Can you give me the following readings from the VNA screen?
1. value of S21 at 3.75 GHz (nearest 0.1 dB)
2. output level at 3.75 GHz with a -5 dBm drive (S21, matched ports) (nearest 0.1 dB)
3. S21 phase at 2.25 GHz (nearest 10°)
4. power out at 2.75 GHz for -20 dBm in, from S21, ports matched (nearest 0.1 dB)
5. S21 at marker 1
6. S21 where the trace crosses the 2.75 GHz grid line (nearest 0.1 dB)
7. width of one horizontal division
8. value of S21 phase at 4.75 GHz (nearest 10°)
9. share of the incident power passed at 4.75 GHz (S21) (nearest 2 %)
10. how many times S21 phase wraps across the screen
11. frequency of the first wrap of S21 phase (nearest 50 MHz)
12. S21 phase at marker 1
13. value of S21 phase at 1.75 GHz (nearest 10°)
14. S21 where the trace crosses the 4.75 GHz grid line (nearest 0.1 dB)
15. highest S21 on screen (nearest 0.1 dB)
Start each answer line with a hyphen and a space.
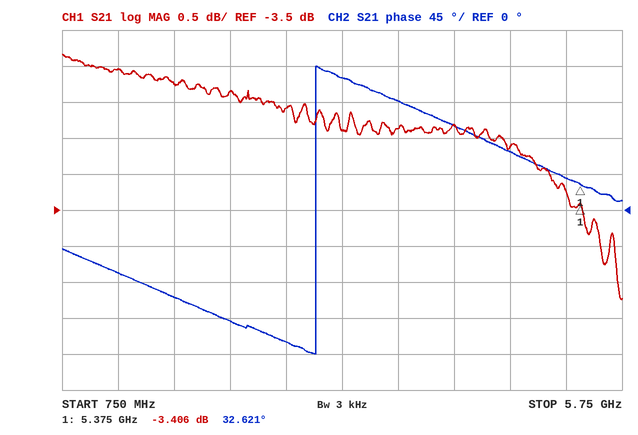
- -2.4 dB
- -7.4 dBm
- -140°
- -22.1 dBm
- -3.406 dB
- -2.1 dB
- 500 MHz
- 70°
- 54 %
- 1
- 3.00 GHz
- 32.621°
- -110°
- -2.6 dB
- -1.3 dB
